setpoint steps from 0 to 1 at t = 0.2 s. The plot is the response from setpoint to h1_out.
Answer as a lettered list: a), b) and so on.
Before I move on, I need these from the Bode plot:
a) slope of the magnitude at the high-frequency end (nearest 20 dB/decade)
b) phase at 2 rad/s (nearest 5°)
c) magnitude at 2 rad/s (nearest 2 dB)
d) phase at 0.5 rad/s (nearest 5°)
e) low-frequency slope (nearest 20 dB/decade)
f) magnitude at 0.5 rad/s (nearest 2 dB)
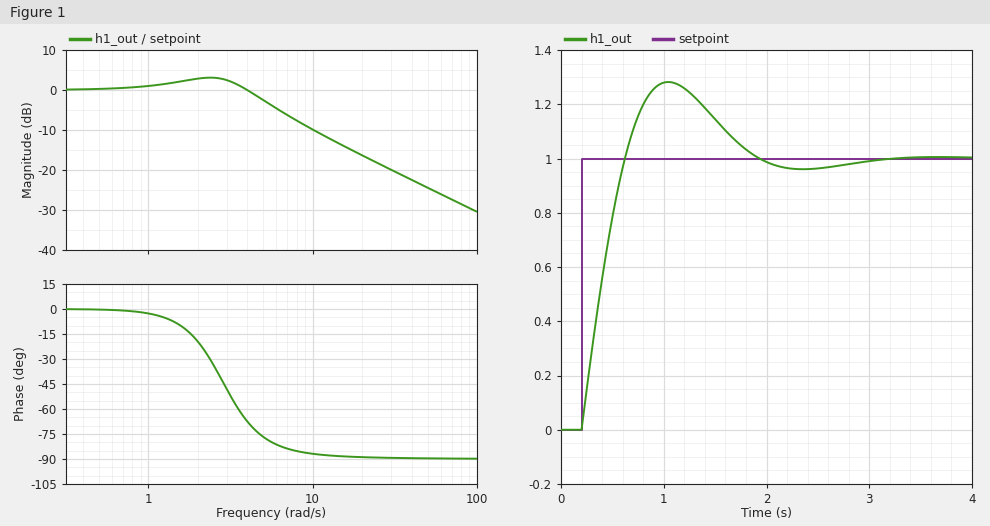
a) -20 dB/decade
b) -20°
c) 2 dB
d) 0°
e) 0 dB/decade
f) 0 dB
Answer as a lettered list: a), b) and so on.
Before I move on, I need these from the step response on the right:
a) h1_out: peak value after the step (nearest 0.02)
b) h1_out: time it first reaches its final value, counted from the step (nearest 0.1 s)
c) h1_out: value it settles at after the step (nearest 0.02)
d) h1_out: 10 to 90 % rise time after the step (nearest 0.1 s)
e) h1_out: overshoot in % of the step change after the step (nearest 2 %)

a) 1.28
b) 0.4 s
c) 1.00
d) 0.3 s
e) 28 %
